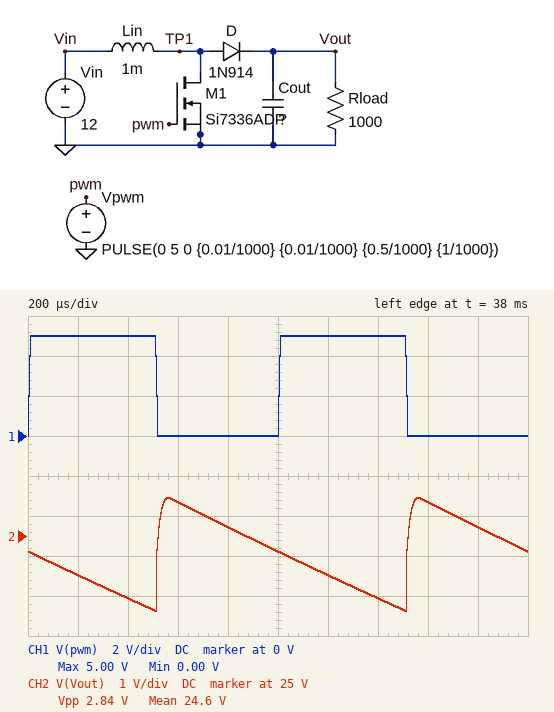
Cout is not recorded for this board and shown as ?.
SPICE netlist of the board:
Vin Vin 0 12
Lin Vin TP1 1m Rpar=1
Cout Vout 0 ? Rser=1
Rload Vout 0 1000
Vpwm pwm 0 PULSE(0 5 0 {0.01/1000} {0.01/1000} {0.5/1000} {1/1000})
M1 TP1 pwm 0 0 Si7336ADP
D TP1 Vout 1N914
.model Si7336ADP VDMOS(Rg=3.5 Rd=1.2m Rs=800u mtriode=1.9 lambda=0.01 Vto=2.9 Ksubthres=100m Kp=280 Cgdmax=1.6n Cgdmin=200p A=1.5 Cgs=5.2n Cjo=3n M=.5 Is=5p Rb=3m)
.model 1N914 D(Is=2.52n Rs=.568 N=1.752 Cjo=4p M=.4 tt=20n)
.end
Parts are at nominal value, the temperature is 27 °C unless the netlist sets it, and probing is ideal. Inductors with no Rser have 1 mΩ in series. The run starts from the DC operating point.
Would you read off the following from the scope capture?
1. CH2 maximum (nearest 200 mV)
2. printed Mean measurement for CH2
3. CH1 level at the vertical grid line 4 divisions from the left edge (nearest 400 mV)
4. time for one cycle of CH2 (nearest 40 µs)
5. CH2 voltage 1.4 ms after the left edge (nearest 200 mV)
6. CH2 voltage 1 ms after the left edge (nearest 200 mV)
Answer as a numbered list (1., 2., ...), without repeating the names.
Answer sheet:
1. 26.0 V
2. 24.6 V
3. 0 V
4. 1.00 ms
5. 23.4 V
6. 24.6 V
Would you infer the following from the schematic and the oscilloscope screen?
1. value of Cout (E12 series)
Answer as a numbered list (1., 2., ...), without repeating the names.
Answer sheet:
1. 8.2 µF
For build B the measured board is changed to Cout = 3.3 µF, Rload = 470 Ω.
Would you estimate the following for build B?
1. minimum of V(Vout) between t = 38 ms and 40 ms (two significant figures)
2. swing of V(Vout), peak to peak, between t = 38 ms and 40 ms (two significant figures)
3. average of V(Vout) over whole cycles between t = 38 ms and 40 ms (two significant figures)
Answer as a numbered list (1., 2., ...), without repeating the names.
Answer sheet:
1. 15 V
2. 11 V
3. 21 V
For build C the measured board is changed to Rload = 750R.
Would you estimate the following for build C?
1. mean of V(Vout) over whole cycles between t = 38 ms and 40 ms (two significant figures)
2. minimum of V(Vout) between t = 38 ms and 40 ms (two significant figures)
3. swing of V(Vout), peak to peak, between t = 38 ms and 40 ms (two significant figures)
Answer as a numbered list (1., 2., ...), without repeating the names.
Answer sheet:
1. 24 V
2. 22 V
3. 3.7 V
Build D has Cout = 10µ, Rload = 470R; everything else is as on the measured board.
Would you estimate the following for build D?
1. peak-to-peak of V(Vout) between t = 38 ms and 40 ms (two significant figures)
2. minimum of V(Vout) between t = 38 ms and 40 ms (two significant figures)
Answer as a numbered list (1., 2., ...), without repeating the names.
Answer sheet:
1. 4.6 V
2. 21 V
